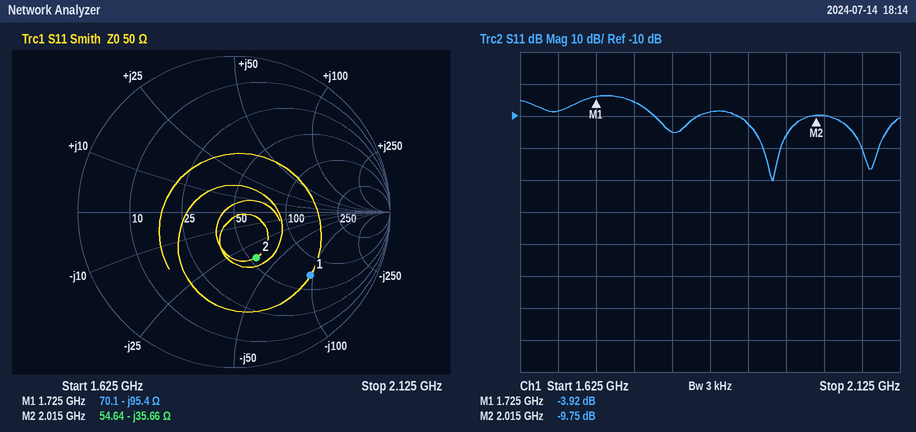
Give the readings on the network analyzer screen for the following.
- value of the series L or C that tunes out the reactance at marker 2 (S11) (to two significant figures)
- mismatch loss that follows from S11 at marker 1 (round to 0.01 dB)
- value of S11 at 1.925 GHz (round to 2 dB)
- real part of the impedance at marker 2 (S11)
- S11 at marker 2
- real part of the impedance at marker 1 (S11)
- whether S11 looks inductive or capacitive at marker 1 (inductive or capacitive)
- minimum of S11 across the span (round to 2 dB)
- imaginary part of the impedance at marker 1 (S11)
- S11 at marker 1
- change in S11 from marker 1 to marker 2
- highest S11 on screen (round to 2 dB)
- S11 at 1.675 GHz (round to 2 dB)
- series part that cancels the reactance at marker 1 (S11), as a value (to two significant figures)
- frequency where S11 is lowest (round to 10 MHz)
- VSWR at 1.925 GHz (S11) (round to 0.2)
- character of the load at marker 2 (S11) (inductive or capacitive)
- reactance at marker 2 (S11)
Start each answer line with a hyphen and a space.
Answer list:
- 2.8 nH
- 2.26 dB
- -12 dB
- 54.64 Ω
- -9.75 dB
- 70.1 Ω
- capacitive
- -30 dB
- -95.4 Ω
- -3.92 dB
- -5.83 dB
- -4 dB
- -8 dB
- 8.8 nH
- 1.96 GHz
- 1.6
- capacitive
- -35.66 Ω
